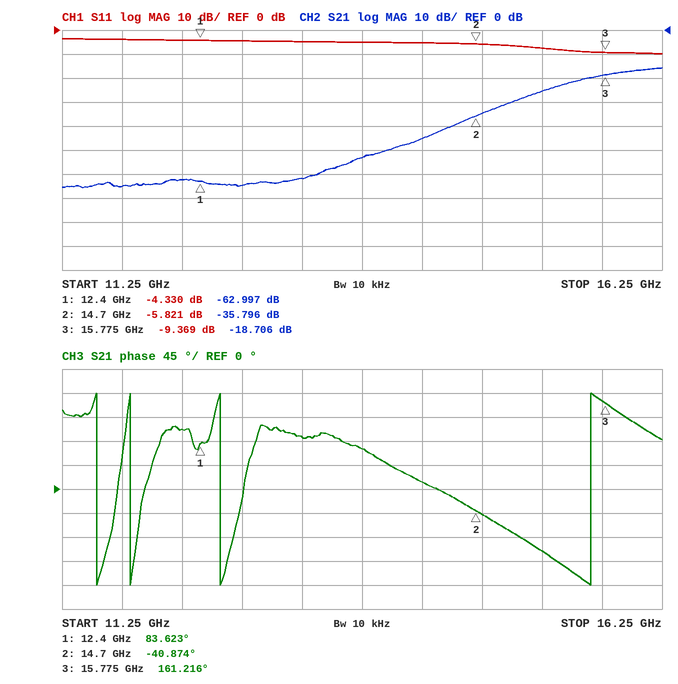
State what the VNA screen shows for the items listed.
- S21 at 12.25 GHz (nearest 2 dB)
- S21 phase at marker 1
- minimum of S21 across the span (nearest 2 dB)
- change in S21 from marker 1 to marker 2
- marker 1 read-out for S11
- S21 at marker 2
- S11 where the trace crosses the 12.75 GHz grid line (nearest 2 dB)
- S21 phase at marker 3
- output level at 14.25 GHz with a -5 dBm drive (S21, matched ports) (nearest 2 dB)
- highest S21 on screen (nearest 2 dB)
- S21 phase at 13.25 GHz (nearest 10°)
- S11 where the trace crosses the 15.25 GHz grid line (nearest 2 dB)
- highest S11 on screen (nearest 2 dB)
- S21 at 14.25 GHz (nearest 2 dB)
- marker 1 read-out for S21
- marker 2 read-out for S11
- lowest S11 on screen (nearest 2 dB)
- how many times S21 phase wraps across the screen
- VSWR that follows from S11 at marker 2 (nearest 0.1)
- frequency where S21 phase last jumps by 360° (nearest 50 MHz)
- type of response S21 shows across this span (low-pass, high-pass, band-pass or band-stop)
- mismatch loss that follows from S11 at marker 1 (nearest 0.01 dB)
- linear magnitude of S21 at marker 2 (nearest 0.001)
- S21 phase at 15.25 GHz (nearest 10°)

-62 dB
83.623°
-66 dB
27.201 dB
-4.330 dB
-35.796 dB
-4 dB
161.216°
-50 dBm
-16 dB
100°
-8 dB
-4 dB
-46 dB
-62.997 dB
-5.821 dB
-10 dB
4
3.1
15.65 GHz
high-pass
2.00 dB
0.016
-120°
